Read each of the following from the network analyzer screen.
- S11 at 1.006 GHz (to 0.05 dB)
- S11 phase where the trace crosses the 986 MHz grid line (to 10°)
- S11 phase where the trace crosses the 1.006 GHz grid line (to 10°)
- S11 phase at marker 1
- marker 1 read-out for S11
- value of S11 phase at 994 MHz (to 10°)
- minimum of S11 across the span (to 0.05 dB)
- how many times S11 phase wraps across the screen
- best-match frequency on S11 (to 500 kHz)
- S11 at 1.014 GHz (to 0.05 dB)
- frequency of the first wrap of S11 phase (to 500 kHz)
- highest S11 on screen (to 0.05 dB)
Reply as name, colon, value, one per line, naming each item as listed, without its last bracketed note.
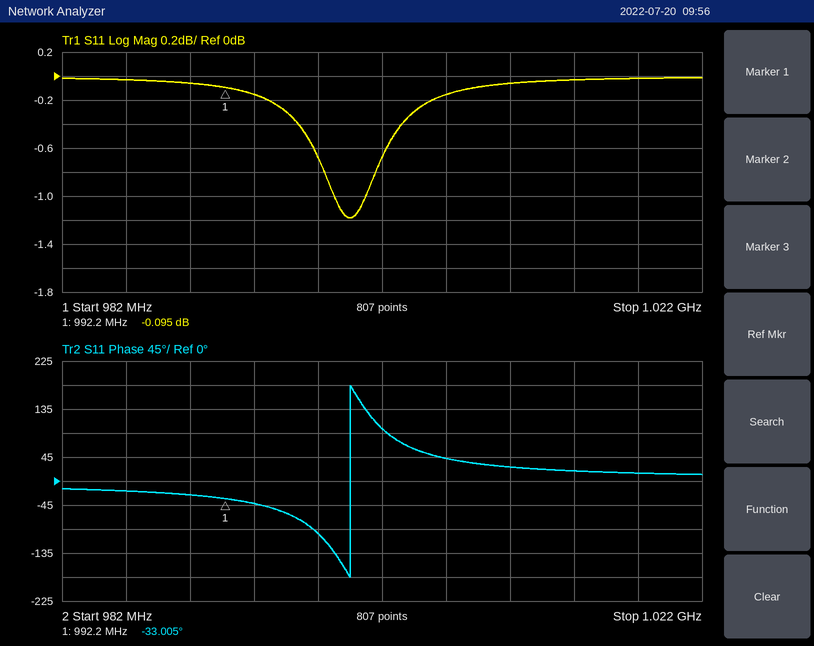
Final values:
S11 at 1.006 GHz: -0.15 dB
S11 phase where the trace crosses the 986 MHz grid line: -20°
S11 phase where the trace crosses the 1.006 GHz grid line: 40°
S11 phase at marker 1: -33.005°
marker 1 read-out for S11: -0.095 dB
value of S11 phase at 994 MHz: -40°
minimum of S11 across the span: -1.20 dB
how many times S11 phase wraps across the screen: 1
best-match frequency on S11: 1.0000 GHz
S11 at 1.014 GHz: -0.05 dB
frequency of the first wrap of S11 phase: 1.0000 GHz
highest S11 on screen: 0.00 dB
